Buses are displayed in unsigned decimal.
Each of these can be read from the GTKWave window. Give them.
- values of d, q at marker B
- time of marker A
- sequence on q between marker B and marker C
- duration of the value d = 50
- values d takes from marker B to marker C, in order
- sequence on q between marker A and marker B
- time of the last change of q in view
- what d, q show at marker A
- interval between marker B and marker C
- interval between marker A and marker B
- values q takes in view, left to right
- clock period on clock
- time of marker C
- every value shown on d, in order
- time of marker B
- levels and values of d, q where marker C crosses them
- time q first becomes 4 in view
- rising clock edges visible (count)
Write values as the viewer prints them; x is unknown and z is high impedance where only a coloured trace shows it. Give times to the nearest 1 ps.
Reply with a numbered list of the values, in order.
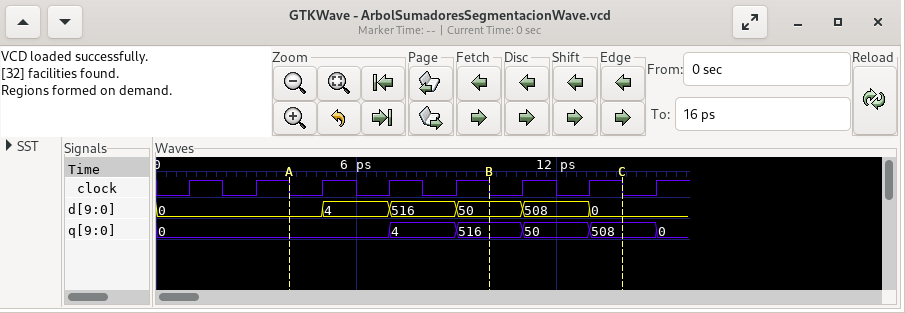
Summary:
1. d=50, q=516
2. 4 ps
3. 516, 50, 508
4. 2 ps
5. 50, 508, 0
6. 0, 4, 516
7. 15 ps
8. d=0, q=0
9. 4 ps
10. 6 ps
11. 0, 4, 516, 50, 508, 0
12. 2 ps
13. 14 ps
14. 0, 4, 516, 50, 508, 0
15. 10 ps
16. d=0, q=508
17. 7 ps
18. 8
